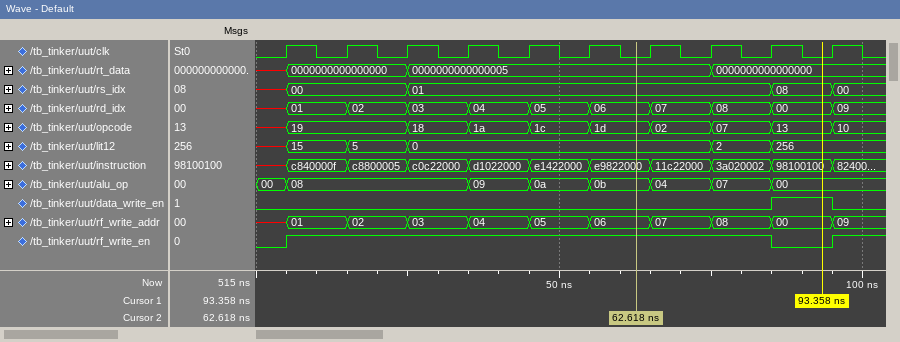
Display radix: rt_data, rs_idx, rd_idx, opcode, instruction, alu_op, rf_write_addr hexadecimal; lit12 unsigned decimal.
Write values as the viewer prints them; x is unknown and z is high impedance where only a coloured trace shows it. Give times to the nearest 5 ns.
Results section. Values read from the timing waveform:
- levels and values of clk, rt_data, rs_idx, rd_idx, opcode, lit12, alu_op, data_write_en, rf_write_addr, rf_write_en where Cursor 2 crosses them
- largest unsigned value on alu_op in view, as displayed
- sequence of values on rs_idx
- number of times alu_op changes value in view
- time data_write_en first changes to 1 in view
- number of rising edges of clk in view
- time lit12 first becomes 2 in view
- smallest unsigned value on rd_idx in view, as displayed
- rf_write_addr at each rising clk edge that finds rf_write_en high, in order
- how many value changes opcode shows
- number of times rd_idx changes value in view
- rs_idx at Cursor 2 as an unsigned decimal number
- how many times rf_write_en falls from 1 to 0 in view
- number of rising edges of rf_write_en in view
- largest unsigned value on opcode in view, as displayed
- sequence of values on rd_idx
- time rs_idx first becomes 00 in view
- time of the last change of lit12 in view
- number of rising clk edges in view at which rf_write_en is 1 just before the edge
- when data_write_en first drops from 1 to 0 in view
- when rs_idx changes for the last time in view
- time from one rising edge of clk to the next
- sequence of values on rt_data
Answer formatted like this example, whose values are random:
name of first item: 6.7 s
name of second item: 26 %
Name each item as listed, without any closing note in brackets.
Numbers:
levels and values of clk, rt_data, rs_idx, rd_idx, opcode, lit12, alu_op, data_write_en, rf_write_addr, rf_write_en where Cursor 2 crosses them: clk=0, rt_data=0000000000000005, rs_idx=01, rd_idx=06, opcode=1d, lit12=0, alu_op=0b, data_write_en=0, rf_write_addr=06, rf_write_en=1
largest unsigned value on alu_op in view, as displayed: 0b
sequence of values on rs_idx: x, 00, 01, 08, 00
number of times alu_op changes value in view: 7
time data_write_en first changes to 1 in view: 85 ns
number of rising edges of clk in view: 10
time lit12 first becomes 2 in view: 75 ns
smallest unsigned value on rd_idx in view, as displayed: 00
rf_write_addr at each rising clk edge that finds rf_write_en high, in order: 01, 02, 03, 04, 05, 06, 07, 08
how many value changes opcode shows: 9
number of times rd_idx changes value in view: 10
rs_idx at Cursor 2 as an unsigned decimal number: 1
how many times rf_write_en falls from 1 to 0 in view: 1
number of rising edges of rf_write_en in view: 2
largest unsigned value on opcode in view, as displayed: 1d
sequence of values on rd_idx: x, 01, 02, 03, 04, 05, 06, 07, 08, 00, 09
time rs_idx first becomes 00 in view: 5 ns
time of the last change of lit12 in view: 85 ns
number of rising clk edges in view at which rf_write_en is 1 just before the edge: 8
when data_write_en first drops from 1 to 0 in view: 95 ns
when rs_idx changes for the last time in view: 95 ns
time from one rising edge of clk to the next: 10 ns
sequence of values on rt_data: x, 0000000000000000, 0000000000000005, 0000000000000000
